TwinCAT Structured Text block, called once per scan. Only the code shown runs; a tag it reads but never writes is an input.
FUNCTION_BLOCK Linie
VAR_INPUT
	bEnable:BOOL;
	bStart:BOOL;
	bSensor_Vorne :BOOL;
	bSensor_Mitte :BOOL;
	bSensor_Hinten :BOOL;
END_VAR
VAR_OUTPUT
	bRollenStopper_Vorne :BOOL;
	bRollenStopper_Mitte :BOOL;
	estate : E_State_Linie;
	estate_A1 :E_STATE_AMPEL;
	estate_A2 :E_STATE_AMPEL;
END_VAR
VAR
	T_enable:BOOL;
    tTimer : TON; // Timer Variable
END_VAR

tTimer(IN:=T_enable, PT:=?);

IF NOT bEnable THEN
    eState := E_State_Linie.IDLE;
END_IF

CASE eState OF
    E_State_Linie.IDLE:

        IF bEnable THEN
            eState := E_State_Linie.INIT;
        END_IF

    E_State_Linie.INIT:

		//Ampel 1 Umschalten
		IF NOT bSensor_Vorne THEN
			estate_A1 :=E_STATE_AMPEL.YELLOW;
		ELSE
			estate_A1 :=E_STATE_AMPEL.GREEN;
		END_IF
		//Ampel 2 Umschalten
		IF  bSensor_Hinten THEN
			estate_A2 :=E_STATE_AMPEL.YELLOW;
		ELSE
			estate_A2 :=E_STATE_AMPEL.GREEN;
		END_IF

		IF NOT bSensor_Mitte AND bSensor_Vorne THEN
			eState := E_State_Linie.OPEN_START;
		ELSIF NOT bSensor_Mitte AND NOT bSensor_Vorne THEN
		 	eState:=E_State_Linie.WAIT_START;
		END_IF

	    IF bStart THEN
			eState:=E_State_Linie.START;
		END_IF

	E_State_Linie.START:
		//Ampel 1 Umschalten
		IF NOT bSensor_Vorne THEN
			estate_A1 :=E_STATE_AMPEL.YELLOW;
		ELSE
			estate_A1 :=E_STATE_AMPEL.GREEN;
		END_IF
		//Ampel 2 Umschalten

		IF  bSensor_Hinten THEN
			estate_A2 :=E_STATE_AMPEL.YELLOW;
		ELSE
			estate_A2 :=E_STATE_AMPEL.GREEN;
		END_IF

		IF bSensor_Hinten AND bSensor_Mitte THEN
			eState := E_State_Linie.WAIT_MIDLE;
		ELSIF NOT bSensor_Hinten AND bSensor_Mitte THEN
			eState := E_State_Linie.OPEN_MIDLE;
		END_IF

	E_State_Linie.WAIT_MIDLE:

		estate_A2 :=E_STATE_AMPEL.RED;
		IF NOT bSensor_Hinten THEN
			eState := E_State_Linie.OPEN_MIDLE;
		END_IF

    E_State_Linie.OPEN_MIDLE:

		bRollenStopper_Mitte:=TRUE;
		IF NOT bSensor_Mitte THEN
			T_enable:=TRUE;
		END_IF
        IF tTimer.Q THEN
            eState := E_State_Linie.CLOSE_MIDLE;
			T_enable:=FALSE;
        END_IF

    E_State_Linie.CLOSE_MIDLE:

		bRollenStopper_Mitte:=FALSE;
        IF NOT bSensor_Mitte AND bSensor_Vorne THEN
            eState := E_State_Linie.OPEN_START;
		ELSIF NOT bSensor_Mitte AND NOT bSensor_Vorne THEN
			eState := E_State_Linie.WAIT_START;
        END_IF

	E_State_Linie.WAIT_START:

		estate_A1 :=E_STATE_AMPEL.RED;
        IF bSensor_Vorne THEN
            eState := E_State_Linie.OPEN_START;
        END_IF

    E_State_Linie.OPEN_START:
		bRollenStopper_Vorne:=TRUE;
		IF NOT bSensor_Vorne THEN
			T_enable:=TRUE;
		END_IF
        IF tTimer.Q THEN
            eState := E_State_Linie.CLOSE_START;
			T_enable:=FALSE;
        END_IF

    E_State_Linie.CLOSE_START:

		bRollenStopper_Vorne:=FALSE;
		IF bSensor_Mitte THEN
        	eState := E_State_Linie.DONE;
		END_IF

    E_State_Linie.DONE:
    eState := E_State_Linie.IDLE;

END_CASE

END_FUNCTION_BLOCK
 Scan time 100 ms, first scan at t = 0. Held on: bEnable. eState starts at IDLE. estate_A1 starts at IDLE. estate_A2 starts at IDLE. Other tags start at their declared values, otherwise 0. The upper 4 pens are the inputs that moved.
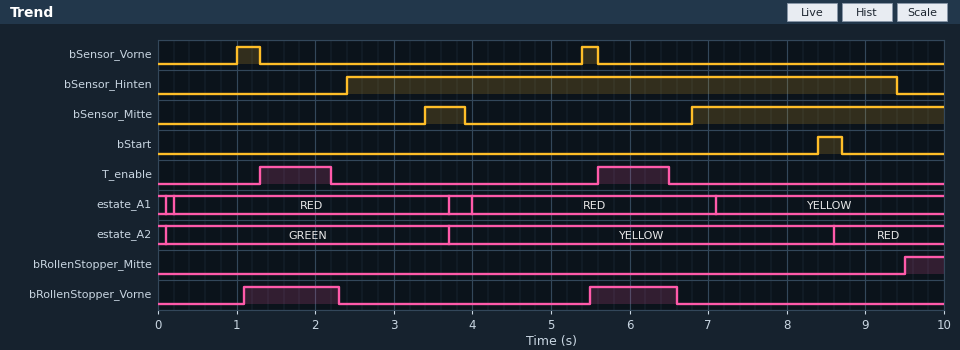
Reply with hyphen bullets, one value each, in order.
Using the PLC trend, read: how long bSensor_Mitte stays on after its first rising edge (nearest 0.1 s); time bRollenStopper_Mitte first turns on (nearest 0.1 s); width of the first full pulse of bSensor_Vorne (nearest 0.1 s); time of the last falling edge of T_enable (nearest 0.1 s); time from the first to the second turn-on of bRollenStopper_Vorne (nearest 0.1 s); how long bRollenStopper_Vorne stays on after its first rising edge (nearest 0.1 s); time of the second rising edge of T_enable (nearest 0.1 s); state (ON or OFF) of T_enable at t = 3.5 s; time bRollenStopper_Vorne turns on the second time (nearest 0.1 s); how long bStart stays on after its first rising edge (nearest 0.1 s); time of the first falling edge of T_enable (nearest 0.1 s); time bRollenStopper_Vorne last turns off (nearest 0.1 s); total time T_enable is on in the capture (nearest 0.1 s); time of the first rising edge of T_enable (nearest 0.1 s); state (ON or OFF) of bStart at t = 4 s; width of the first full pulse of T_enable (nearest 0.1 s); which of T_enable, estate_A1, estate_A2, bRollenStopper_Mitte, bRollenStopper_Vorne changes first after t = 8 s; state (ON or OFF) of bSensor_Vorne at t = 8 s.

- 0.5 s
- 9.5 s
- 0.3 s
- 6.5 s
- 4.4 s
- 1.2 s
- 5.6 s
- OFF
- 5.5 s
- 0.3 s
- 2.2 s
- 6.6 s
- 1.8 s
- 1.3 s
- OFF
- 0.9 s
- estate_A2
- OFF
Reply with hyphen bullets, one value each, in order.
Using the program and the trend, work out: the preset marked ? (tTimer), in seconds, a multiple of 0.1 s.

- 0.8 s
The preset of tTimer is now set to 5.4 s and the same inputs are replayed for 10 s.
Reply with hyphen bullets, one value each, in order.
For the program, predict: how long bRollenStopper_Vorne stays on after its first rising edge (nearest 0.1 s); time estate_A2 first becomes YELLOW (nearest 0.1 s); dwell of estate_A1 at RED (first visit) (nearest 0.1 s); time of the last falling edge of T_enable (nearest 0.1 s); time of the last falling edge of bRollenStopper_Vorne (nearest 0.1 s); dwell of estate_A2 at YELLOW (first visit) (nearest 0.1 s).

- 5.8 s
- 7.2 s
- 7.0 s
- 6.8 s
- 6.9 s
- 1.4 s
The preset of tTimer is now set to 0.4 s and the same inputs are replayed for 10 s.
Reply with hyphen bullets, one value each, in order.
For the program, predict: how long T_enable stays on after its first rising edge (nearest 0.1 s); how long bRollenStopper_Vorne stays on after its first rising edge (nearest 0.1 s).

- 0.5 s
- 0.8 s
